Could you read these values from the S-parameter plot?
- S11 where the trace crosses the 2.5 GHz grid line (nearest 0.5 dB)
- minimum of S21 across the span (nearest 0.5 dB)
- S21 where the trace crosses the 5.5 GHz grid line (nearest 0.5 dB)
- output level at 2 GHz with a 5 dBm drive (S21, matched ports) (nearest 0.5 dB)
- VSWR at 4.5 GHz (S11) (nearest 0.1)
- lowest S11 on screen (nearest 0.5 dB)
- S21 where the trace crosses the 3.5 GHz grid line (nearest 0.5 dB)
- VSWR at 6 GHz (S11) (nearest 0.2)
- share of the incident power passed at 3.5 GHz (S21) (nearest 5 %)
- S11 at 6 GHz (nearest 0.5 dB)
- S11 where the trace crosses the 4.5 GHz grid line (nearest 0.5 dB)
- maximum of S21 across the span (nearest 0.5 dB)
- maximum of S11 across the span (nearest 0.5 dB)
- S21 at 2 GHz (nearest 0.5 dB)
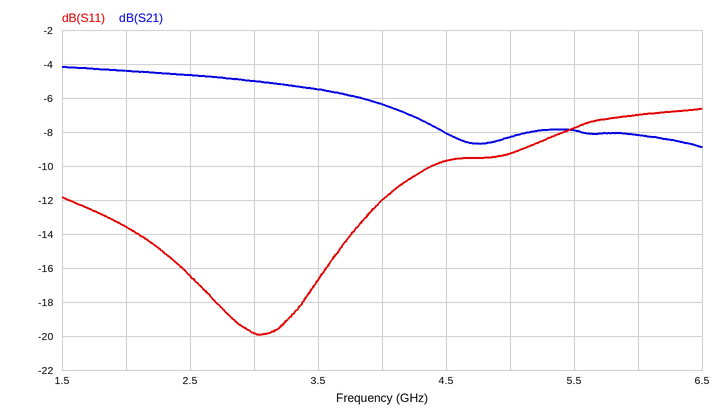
-16.5 dB
-9.0 dB
-8.0 dB
0.5 dBm
2.0
-20.0 dB
-5.5 dB
2.6
30 %
-7.0 dB
-9.5 dB
-4.0 dB
-6.5 dB
-4.5 dB
